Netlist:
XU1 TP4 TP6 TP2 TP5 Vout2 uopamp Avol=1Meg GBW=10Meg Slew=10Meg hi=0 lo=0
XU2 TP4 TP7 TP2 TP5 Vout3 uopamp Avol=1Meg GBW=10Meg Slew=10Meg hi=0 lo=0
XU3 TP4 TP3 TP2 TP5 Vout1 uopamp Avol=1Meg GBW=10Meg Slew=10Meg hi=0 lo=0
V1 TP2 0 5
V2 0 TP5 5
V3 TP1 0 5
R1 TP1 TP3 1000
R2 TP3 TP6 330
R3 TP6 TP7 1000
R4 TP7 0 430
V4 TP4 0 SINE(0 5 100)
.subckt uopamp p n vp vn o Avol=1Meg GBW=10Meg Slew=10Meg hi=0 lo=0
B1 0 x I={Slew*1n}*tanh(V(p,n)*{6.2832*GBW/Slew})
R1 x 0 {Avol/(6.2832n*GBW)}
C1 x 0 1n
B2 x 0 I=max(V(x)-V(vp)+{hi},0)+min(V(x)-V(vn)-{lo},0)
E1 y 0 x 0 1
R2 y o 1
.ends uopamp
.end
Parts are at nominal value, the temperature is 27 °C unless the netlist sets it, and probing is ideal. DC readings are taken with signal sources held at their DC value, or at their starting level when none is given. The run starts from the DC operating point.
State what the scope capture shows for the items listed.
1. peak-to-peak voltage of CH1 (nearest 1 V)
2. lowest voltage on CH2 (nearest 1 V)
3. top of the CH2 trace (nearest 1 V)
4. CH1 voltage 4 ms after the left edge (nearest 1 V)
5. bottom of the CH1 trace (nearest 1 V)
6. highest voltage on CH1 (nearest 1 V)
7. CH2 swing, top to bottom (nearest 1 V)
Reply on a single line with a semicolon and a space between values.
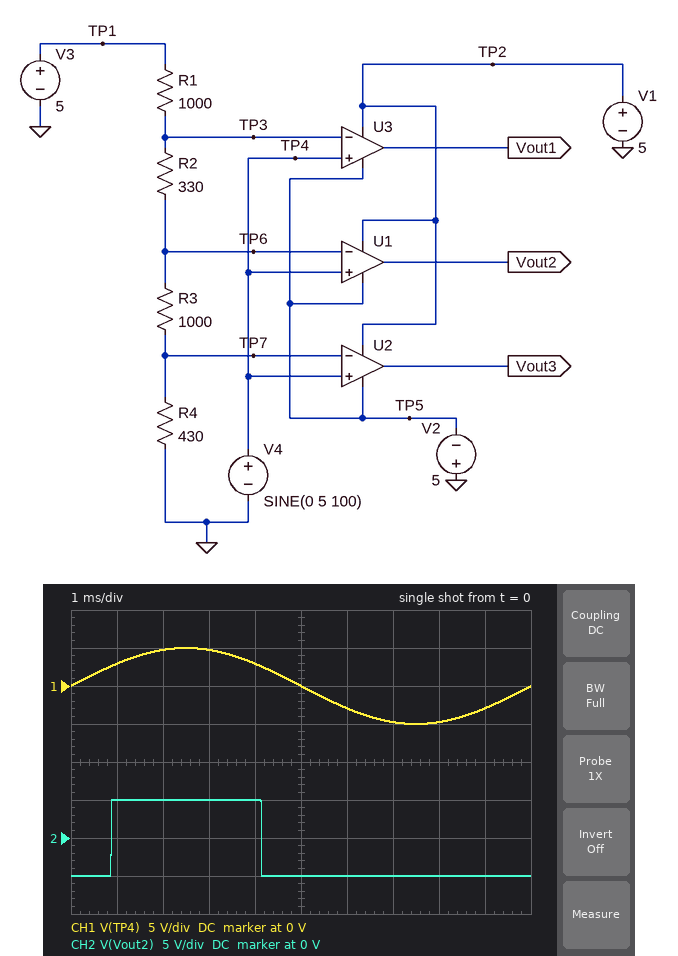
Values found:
10 V; -5 V; 5 V; 3 V; -5 V; 5 V; 10 V
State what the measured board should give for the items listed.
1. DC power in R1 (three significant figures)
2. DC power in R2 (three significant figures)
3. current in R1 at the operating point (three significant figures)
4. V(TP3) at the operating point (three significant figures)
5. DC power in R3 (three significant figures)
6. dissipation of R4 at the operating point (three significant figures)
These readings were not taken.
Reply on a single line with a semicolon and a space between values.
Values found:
3.28 mW; 1.08 mW; 1.81 mA; 3.19 V; 3.28 mW; 1.41 mW
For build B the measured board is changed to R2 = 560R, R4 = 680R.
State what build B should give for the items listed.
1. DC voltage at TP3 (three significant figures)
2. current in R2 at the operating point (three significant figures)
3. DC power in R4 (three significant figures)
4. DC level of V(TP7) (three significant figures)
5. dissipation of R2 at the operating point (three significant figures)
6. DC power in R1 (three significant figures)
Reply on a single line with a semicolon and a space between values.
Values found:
3.46 V; 1.54 mA; 1.62 mW; 1.05 V; 1.33 mW; 2.38 mW
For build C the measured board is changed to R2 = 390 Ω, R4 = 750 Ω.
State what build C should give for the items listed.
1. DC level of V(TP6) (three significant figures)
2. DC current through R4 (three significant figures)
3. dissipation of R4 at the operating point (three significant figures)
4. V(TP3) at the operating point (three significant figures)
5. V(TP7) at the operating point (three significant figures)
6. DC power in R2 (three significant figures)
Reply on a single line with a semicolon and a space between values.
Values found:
2.79 V; 1.59 mA; 1.90 mW; 3.41 V; 1.19 V; 989 µW
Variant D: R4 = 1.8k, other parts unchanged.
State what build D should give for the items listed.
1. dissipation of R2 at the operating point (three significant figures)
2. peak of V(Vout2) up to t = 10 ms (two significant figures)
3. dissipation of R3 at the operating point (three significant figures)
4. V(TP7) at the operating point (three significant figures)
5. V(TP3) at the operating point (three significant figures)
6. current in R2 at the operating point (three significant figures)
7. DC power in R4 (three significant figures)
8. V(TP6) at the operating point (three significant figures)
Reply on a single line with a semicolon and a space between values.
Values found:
484 µW; 5.0 V; 1.47 mW; 2.18 V; 3.79 V; 1.21 mA; 2.64 mW; 3.39 V
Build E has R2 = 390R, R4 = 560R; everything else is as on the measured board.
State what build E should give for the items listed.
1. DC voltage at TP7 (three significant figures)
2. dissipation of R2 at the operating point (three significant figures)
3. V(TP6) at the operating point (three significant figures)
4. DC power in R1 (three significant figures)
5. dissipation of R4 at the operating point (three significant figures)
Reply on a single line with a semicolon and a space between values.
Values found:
949 mV; 1.12 mW; 2.64 V; 2.87 mW; 1.61 mW
